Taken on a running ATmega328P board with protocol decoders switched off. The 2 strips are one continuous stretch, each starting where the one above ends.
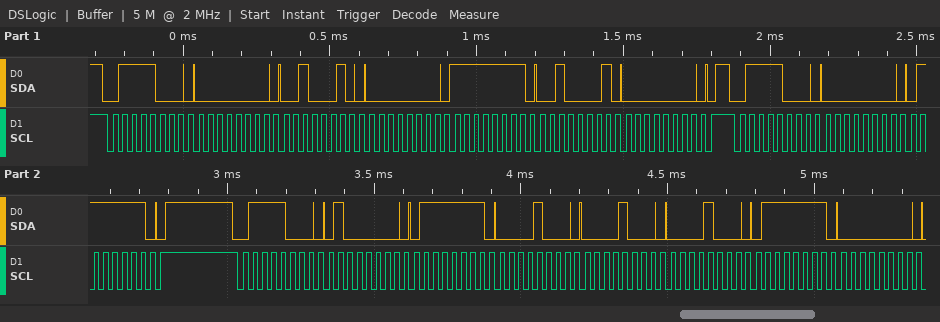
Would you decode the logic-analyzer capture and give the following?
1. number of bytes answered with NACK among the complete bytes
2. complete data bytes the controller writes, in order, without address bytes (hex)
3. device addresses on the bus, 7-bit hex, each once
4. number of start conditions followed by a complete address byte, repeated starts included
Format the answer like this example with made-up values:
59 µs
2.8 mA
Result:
0
00 22 00 FF 21 00 00 7F 40 7F 08 08 08 7F 00
0x3C
3
